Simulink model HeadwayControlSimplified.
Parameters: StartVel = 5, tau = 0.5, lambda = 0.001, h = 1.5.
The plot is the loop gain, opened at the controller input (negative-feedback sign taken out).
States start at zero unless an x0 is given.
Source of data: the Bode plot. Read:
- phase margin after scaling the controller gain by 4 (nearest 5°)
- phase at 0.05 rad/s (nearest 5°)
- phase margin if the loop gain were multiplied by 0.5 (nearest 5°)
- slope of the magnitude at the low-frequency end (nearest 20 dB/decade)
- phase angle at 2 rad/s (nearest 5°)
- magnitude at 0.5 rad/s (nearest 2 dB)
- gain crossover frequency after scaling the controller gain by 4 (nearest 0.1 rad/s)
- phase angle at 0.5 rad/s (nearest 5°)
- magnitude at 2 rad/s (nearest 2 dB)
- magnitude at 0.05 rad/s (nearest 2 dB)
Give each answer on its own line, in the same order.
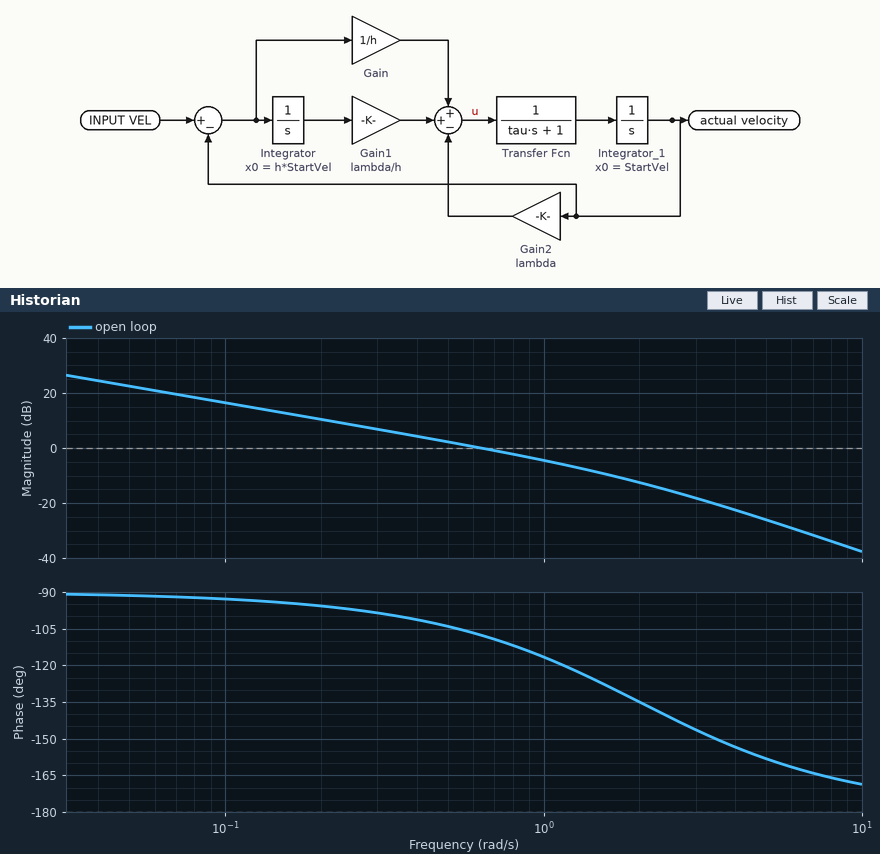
45°
-90°
80°
-20 dB/decade
-135°
2 dB
1.9 rad/s
-105°
-12 dB
22 dB
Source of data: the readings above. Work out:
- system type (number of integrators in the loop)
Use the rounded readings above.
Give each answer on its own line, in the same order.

1
